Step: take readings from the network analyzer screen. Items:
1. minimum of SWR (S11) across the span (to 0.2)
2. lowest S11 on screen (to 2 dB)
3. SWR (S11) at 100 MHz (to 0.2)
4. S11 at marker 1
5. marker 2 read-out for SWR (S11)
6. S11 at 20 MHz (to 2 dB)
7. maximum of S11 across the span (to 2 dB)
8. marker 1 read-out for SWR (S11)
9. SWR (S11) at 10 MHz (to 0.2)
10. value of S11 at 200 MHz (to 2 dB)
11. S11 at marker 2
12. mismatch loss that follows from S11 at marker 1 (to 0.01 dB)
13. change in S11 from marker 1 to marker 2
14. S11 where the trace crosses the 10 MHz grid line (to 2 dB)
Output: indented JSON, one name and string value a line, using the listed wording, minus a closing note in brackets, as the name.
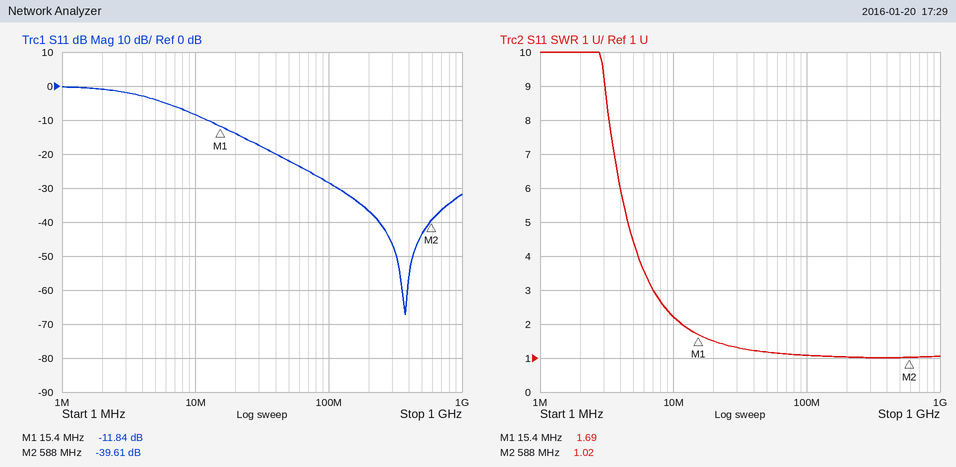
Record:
{
  "minimum of SWR (S11) across the span": "1.0",
  "lowest S11 on screen": "-68 dB",
  "SWR (S11) at 100 MHz": "1.0",
  "S11 at marker 1": "-11.84 dB",
  "marker 2 read-out for SWR": "1.02",
  "S11 at 20 MHz": "-14 dB",
  "maximum of S11 across the span": "0 dB",
  "marker 1 read-out for SWR": "1.69",
  "SWR (S11) at 10 MHz": "2.2",
  "value of S11 at 200 MHz": "-36 dB",
  "S11 at marker 2": "-39.61 dB",
  "mismatch loss that follows from S11 at marker 1": "0.29 dB",
  "change in S11 from marker 1 to marker 2": "-27.77 dB",
  "S11 where the trace crosses the 10 MHz grid line": "-8 dB"
}
